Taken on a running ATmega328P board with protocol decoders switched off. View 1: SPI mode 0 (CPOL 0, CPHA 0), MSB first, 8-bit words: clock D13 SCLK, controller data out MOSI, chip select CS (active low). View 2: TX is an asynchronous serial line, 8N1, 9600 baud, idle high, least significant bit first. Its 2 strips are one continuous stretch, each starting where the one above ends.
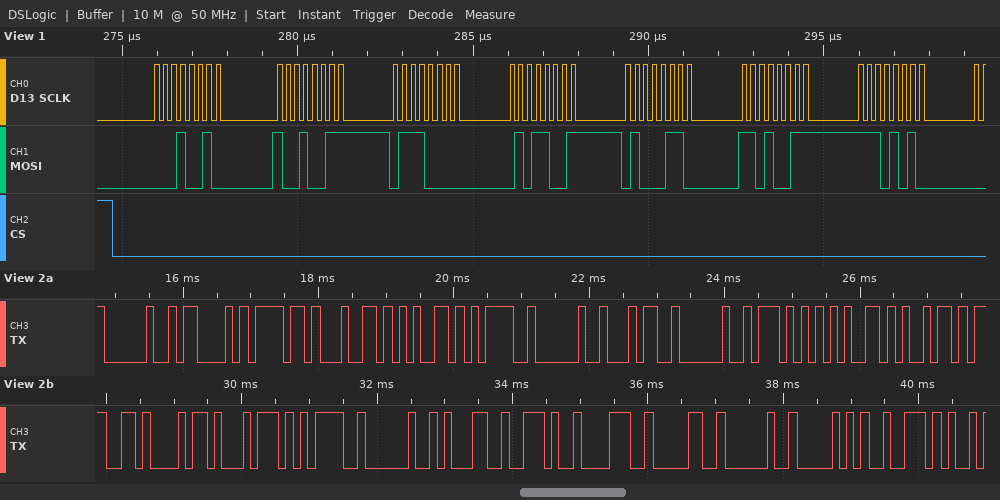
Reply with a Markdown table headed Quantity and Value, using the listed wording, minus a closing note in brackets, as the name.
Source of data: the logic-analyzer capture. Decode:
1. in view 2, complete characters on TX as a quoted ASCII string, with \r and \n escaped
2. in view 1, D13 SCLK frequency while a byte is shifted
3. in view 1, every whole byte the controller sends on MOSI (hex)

| Quantity | Value |
|---|---|
| in view 2, complete characters on TX as a quoted ASCII string, with \r and \n escaped | " Code= 4 Weight= 1.80 Pr" |
| in view 1, D13 SCLK frequency while a byte is shifted | 4 MHz |
| in view 1, every whole byte the controller sends on MOSI | 12 93 70 59 46 D3 EA |
